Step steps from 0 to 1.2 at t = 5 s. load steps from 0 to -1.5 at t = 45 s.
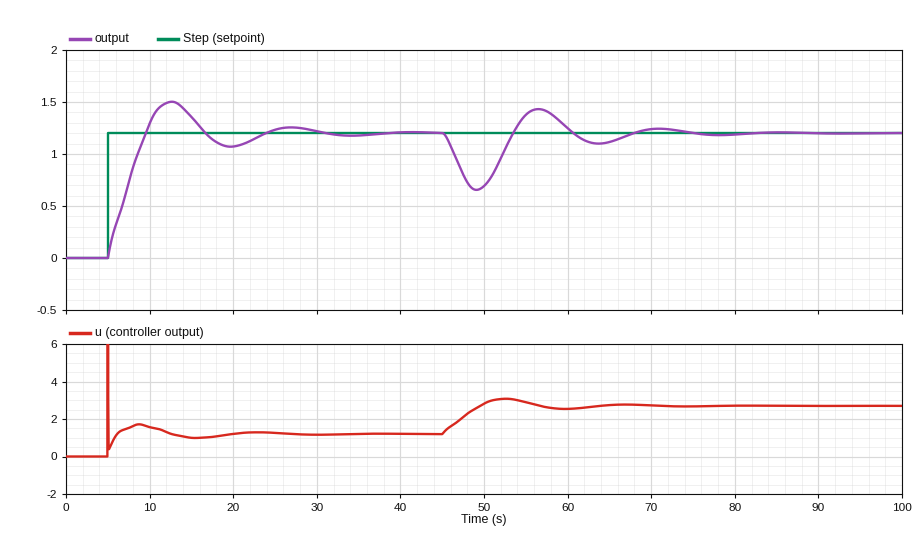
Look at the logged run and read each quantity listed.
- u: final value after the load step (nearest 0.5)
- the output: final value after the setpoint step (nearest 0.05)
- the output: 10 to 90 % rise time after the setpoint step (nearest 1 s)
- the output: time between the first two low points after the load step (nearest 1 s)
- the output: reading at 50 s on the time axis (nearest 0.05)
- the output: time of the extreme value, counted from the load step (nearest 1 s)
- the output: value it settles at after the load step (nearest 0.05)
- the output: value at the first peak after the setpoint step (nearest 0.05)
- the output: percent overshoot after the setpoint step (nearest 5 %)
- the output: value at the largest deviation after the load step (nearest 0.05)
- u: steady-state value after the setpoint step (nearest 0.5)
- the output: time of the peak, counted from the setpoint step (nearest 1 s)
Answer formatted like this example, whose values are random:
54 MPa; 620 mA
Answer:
2.5; 1.20; 4 s; 15 s; 0.70; 4 s; 1.20; 1.50; 25 %; 0.65; 1.0; 8 s
